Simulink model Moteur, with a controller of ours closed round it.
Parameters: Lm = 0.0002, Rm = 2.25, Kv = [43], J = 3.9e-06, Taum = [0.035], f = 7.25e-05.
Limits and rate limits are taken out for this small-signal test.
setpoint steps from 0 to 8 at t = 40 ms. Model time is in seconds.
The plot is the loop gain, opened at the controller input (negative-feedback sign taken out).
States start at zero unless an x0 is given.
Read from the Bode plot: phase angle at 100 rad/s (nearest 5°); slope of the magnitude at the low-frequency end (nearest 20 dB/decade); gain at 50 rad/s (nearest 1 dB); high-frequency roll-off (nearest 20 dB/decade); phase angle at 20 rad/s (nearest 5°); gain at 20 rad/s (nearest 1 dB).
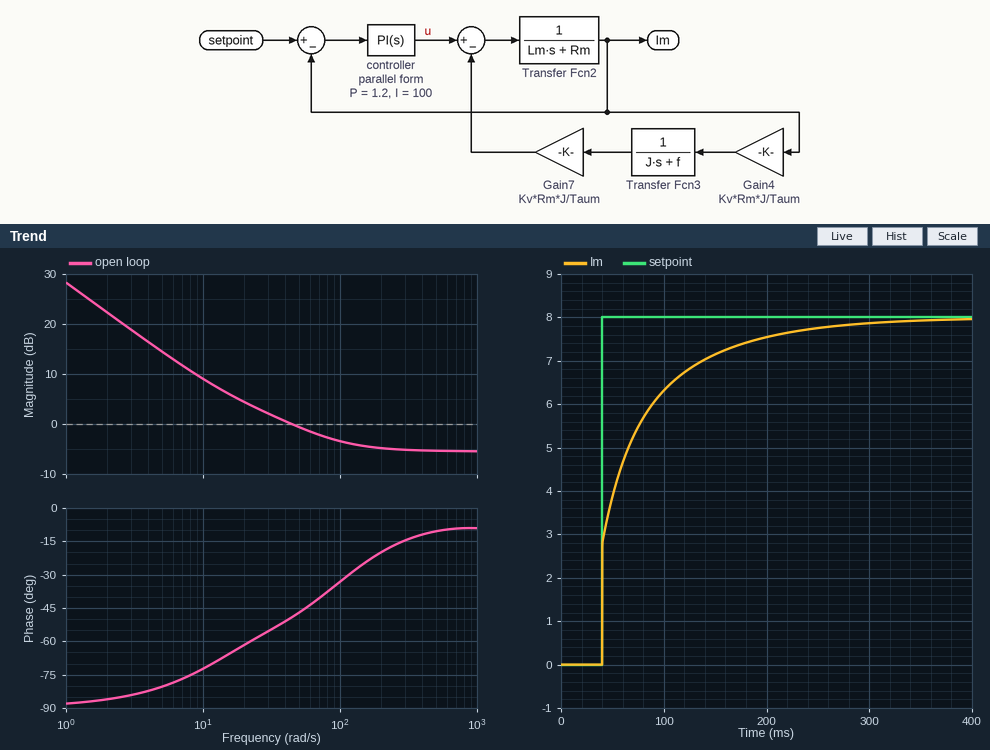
-35°
-20 dB/decade
-1 dB
0 dB/decade
-60°
4 dB
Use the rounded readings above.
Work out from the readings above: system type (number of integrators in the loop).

1
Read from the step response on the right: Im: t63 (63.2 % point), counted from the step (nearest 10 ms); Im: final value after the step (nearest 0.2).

30 ms
8.0
